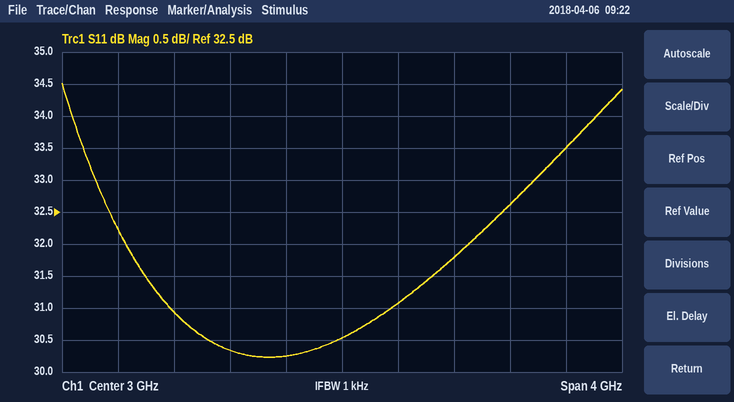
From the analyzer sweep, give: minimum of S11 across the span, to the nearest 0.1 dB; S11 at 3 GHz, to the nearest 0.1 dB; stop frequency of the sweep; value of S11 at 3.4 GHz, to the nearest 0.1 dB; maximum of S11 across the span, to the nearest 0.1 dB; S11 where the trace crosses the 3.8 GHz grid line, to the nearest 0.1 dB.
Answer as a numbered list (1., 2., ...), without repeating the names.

1. 30.2 dB
2. 30.5 dB
3. 5 GHz
4. 31.1 dB
5. 34.5 dB
6. 31.8 dB
